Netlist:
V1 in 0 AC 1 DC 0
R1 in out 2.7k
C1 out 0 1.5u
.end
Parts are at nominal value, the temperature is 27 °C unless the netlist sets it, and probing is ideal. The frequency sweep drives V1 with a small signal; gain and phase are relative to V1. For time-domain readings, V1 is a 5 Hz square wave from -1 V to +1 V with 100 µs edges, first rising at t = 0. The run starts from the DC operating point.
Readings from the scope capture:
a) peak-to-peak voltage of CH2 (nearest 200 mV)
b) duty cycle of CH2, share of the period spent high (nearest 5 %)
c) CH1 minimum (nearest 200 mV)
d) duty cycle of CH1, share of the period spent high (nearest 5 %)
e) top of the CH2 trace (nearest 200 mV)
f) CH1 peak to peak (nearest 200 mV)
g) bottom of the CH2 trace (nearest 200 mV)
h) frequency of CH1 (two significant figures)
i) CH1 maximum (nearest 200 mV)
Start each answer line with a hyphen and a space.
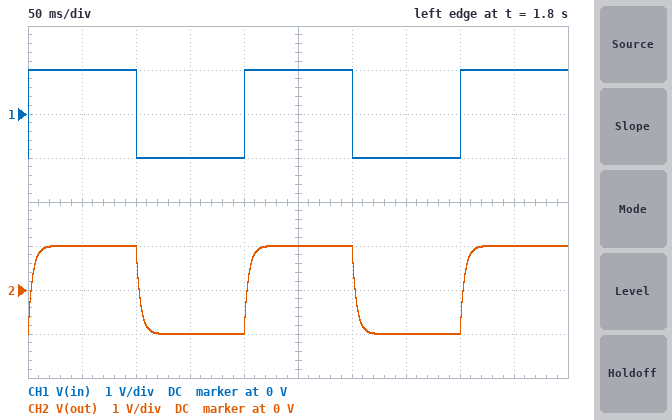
- 2.0 V
- 50 %
- -1.0 V
- 50 %
- 1.0 V
- 2.0 V
- -1.0 V
- 5.0 Hz
- 1.0 V
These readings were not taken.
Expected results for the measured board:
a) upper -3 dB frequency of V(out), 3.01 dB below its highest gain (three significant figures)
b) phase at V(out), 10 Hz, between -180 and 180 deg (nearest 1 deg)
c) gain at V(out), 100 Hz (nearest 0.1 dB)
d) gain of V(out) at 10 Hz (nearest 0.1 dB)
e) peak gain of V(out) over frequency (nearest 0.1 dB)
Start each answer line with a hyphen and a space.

- 39.3 Hz
- -14 deg
- -8.7 dB
- -0.3 dB
- 0 dB
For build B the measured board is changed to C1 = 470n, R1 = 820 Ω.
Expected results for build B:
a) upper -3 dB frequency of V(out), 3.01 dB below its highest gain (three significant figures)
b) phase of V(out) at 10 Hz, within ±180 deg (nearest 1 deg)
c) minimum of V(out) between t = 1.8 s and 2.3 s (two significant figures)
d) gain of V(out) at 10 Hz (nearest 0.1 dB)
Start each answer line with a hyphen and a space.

- 413 Hz
- -1 deg
- -1.0 V
- 0 dB
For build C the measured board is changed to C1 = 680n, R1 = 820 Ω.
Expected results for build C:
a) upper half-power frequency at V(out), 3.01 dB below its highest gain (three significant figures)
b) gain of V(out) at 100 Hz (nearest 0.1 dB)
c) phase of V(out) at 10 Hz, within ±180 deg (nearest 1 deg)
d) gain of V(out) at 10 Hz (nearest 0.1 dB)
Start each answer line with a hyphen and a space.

- 285 Hz
- -0.5 dB
- -2 deg
- 0 dB
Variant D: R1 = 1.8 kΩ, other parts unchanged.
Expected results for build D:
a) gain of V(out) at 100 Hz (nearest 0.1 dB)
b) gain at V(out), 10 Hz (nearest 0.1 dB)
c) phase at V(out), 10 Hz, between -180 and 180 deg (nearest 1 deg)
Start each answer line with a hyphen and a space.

- -5.9 dB
- -0.1 dB
- -10 deg
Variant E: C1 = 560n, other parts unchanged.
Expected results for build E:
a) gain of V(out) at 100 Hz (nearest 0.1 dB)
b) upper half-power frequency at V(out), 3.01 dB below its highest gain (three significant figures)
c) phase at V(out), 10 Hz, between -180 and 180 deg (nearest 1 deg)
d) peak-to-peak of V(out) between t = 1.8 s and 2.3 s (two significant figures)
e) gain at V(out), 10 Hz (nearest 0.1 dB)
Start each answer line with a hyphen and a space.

- -2.8 dB
- 105 Hz
- -5 deg
- 2.0 V
- 0 dB
